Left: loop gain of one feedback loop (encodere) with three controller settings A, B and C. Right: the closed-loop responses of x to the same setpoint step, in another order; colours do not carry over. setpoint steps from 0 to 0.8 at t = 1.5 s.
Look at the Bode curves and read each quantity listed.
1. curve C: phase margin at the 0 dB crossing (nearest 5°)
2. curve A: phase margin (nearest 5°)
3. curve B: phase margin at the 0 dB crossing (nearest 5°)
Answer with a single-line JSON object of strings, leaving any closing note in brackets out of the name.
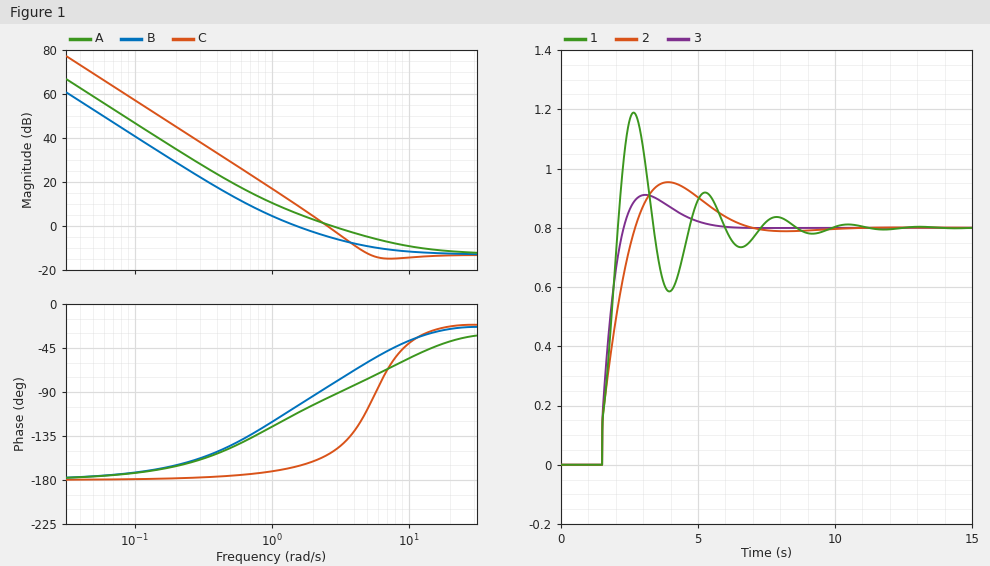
{"curve C: phase margin at the 0 dB crossing": "25°", "curve A: phase margin": "85°", "curve B: phase margin at the 0 dB crossing": "75°"}
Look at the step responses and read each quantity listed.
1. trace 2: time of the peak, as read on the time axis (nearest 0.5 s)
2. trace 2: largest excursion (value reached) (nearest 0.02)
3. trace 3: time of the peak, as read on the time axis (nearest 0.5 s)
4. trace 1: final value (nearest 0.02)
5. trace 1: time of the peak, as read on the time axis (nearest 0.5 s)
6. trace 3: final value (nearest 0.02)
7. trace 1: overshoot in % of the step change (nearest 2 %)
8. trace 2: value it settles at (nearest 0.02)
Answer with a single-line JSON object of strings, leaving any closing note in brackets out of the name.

{"trace 2: time of the peak, as read on the time axis": "4.0 s", "trace 2: largest excursion (value reached)": "0.96", "trace 3: time of the peak, as read on the time axis": "3.0 s", "trace 1: final value": "0.80", "trace 1: time of the peak, as read on the time axis": "2.5 s", "trace 3: final value": "0.80", "trace 1: overshoot in % of the step change": "48 %", "trace 2: value it settles at": "0.80"}
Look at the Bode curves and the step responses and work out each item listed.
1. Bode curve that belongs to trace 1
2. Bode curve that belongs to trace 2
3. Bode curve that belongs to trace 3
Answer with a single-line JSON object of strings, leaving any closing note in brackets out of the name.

{"Bode curve that belongs to trace 1": "C", "Bode curve that belongs to trace 2": "B", "Bode curve that belongs to trace 3": "A"}
